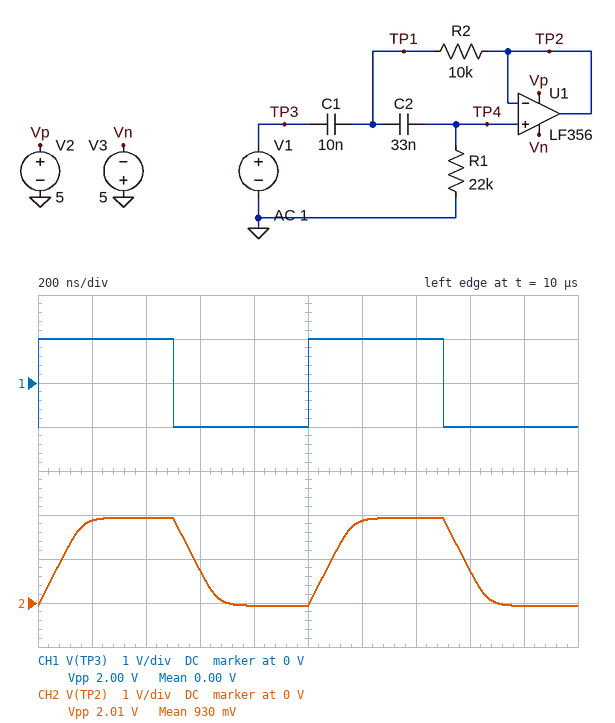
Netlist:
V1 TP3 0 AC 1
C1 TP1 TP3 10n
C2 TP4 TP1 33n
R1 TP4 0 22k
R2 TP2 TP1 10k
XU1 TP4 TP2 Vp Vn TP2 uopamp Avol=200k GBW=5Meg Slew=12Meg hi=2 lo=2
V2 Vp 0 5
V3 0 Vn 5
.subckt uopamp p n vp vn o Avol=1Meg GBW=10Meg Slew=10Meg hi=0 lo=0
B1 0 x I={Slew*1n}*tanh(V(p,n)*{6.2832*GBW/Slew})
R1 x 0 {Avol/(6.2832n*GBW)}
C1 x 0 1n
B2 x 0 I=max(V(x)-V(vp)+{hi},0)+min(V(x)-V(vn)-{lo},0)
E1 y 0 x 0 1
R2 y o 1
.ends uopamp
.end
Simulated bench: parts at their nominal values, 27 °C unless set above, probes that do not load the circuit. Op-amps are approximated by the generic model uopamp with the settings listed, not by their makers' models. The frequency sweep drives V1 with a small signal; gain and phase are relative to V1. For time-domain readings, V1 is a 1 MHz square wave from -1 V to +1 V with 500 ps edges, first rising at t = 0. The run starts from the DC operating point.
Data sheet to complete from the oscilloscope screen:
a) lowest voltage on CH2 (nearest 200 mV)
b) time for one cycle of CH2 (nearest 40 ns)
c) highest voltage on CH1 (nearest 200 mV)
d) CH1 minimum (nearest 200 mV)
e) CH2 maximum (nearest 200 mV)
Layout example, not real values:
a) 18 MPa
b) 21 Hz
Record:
a) 0 V
b) 1.00 µs
c) 1.0 V
d) -1.0 V
e) 2.0 V
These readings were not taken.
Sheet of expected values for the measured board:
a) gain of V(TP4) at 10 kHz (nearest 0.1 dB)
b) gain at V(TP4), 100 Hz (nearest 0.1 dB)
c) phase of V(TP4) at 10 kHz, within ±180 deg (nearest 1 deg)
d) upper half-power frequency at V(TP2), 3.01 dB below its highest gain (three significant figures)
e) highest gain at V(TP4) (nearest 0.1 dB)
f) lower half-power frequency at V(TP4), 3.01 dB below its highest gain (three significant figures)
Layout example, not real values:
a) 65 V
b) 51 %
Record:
a) 0 dB
b) -30.9 dB
c) 5 deg
d) 5.00 MHz
e) 0 dB
f) 676 Hz
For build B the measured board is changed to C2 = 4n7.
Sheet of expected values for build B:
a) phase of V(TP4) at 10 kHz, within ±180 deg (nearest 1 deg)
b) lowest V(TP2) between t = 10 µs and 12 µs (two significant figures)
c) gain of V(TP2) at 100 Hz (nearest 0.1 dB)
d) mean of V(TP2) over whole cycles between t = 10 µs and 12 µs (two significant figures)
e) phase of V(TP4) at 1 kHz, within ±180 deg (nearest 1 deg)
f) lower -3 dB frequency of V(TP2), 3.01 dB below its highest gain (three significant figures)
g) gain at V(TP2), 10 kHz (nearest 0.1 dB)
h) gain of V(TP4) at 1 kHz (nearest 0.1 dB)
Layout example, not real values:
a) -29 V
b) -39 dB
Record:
a) 13 deg
b) -160 mV
c) -47.8 dB
d) 850 mV
e) 123 deg
f) 1.60 kHz
g) 0 dB
h) -8.6 dB
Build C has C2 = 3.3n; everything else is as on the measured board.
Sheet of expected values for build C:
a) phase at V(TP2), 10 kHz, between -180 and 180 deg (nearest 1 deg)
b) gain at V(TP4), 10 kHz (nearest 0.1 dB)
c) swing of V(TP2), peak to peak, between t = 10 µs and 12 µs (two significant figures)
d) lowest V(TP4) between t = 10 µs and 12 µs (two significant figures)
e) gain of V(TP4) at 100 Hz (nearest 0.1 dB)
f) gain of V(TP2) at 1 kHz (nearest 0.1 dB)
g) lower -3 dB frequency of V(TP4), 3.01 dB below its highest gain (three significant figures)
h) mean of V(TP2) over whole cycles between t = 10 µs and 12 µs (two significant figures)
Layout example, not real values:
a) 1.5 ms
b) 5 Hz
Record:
a) 17 deg
b) -0.1 dB
c) 2.0 V
d) -210 mV
e) -50.9 dB
f) -11.7 dB
g) 2.08 kHz
h) 810 mV
